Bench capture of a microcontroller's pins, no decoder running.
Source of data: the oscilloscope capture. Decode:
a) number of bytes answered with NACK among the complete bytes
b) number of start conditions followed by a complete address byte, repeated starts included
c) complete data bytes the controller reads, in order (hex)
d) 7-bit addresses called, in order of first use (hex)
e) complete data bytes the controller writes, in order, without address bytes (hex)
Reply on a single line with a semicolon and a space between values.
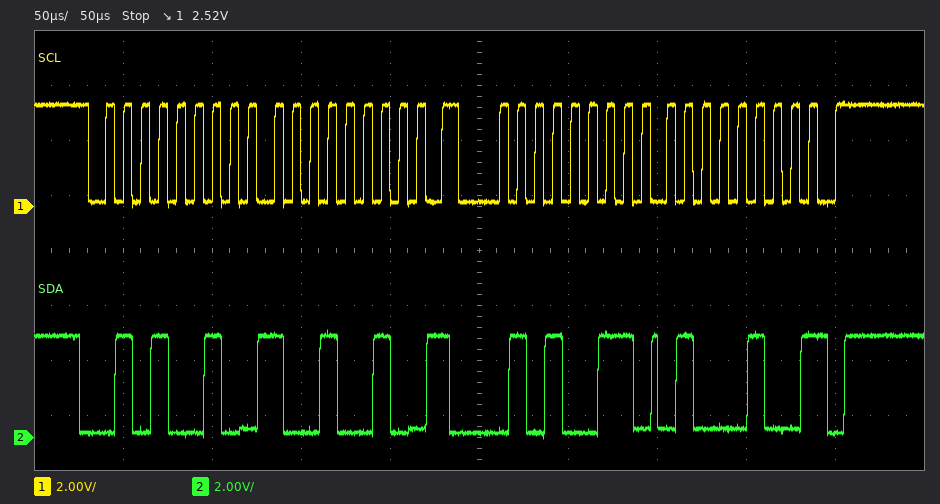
1; 2; 44; 0x29; 92
